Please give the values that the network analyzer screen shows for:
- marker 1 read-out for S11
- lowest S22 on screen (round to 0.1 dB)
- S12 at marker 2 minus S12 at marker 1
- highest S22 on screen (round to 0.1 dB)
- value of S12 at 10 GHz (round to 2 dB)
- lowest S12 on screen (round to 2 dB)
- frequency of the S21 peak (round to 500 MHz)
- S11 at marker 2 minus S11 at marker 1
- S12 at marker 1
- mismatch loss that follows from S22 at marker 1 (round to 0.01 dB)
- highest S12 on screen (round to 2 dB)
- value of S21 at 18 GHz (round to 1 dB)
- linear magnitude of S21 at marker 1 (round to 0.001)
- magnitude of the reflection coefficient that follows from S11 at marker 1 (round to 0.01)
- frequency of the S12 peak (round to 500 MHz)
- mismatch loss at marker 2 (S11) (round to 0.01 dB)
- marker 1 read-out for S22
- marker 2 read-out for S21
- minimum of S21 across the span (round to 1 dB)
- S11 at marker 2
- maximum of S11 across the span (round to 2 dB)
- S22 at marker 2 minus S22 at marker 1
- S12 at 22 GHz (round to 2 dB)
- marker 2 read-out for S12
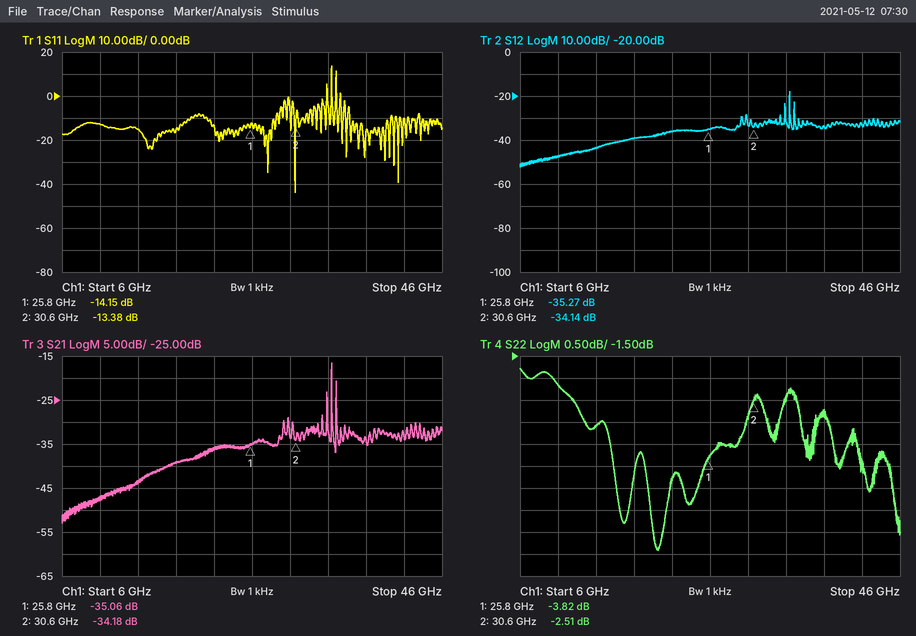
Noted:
-14.15 dB
-5.9 dB
1.13 dB
-1.8 dB
-48 dB
-52 dB
34.5 GHz
0.77 dB
-35.27 dB
2.33 dB
-18 dB
-39 dB
0.018
0.20
34.5 GHz
0.20 dB
-3.82 dB
-34.18 dB
-53 dB
-13.38 dB
14 dB
1.31 dB
-36 dB
-34.14 dB
